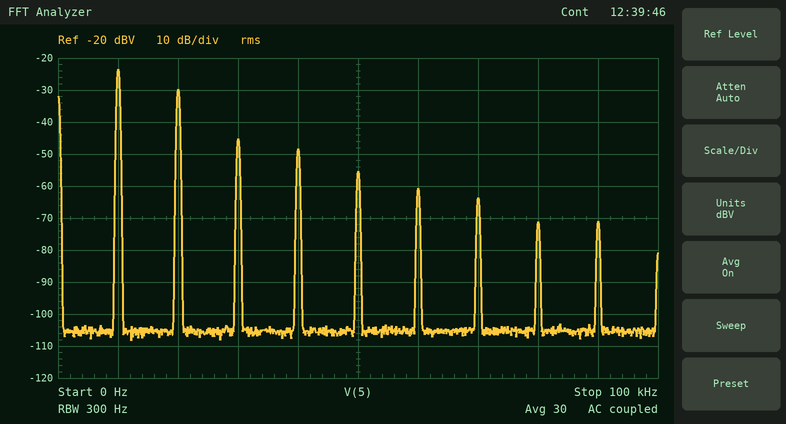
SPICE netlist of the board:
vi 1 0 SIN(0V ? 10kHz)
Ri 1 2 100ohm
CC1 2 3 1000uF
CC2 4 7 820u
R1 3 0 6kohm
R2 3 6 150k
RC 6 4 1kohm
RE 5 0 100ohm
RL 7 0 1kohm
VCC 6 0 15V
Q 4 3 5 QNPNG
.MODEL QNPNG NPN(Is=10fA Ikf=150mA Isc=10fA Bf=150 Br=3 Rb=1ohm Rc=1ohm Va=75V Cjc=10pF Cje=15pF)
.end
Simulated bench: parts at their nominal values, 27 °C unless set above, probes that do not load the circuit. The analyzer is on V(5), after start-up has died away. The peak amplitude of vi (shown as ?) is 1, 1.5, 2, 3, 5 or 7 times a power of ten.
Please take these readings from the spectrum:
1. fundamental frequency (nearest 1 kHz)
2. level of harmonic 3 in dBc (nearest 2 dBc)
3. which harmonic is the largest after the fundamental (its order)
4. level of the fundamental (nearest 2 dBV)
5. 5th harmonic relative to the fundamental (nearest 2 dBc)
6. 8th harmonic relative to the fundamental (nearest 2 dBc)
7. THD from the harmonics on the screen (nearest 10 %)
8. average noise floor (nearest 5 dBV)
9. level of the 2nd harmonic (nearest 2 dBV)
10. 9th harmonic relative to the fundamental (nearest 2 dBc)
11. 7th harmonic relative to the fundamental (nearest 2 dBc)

10 kHz
-22 dBc
2
-24 dBV
-32 dBc
-48 dBc
50 %
-105 dBV
-30 dBV
-48 dBc
-40 dBc
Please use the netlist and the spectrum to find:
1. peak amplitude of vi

300 mV
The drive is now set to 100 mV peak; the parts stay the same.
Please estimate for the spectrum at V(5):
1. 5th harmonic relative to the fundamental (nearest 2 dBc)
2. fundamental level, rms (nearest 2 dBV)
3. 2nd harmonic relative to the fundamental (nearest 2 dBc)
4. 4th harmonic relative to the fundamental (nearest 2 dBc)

-42 dBc
-36 dBV
-8 dBc
-36 dBc
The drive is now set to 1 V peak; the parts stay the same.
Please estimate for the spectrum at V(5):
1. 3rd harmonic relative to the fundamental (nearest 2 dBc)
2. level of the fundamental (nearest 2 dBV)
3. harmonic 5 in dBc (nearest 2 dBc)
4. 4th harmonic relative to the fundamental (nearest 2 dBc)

-28 dBc
-10 dBV
-34 dBc
-22 dBc
